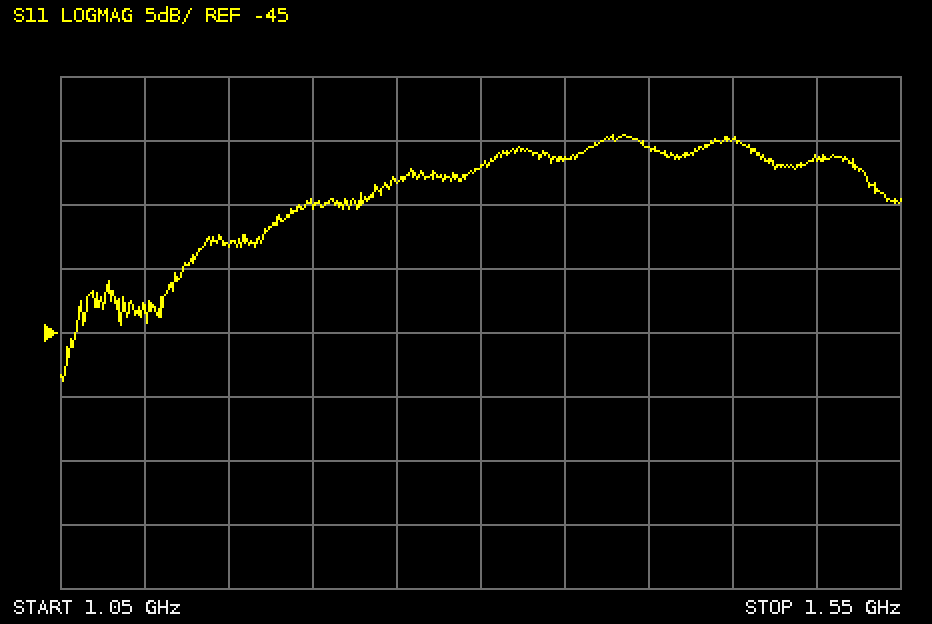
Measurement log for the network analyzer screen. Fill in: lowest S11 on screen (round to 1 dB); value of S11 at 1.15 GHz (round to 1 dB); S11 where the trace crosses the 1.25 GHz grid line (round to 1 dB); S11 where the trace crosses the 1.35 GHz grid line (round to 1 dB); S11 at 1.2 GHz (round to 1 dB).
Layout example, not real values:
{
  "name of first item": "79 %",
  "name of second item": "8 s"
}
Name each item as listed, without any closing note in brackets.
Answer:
{
  "lowest S11 on screen": "-49 dB",
  "value of S11 at 1.15 GHz": "-38 dB",
  "S11 where the trace crosses the 1.25 GHz grid line": "-33 dB",
  "S11 where the trace crosses the 1.35 GHz grid line": "-31 dB",
  "S11 at 1.2 GHz": "-35 dB"
}
